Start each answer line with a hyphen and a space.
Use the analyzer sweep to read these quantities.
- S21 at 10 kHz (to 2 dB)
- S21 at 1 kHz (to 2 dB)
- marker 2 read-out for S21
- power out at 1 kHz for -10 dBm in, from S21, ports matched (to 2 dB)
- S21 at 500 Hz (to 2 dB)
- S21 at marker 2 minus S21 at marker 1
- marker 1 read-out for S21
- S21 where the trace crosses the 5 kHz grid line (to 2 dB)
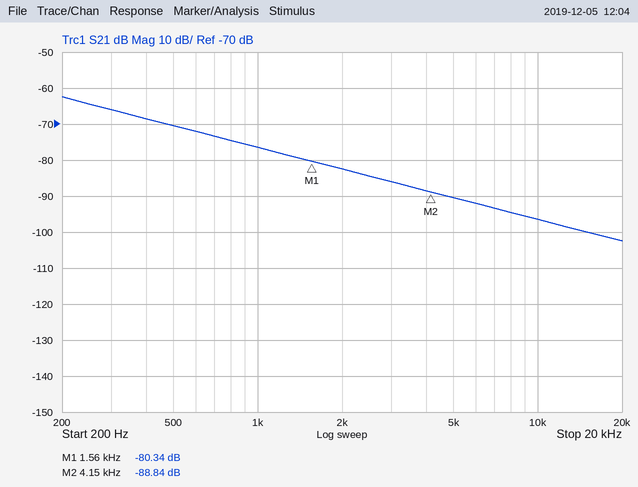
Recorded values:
- -96 dB
- -76 dB
- -88.84 dB
- -86 dBm
- -70 dB
- -8.50 dB
- -80.34 dB
- -90 dB
